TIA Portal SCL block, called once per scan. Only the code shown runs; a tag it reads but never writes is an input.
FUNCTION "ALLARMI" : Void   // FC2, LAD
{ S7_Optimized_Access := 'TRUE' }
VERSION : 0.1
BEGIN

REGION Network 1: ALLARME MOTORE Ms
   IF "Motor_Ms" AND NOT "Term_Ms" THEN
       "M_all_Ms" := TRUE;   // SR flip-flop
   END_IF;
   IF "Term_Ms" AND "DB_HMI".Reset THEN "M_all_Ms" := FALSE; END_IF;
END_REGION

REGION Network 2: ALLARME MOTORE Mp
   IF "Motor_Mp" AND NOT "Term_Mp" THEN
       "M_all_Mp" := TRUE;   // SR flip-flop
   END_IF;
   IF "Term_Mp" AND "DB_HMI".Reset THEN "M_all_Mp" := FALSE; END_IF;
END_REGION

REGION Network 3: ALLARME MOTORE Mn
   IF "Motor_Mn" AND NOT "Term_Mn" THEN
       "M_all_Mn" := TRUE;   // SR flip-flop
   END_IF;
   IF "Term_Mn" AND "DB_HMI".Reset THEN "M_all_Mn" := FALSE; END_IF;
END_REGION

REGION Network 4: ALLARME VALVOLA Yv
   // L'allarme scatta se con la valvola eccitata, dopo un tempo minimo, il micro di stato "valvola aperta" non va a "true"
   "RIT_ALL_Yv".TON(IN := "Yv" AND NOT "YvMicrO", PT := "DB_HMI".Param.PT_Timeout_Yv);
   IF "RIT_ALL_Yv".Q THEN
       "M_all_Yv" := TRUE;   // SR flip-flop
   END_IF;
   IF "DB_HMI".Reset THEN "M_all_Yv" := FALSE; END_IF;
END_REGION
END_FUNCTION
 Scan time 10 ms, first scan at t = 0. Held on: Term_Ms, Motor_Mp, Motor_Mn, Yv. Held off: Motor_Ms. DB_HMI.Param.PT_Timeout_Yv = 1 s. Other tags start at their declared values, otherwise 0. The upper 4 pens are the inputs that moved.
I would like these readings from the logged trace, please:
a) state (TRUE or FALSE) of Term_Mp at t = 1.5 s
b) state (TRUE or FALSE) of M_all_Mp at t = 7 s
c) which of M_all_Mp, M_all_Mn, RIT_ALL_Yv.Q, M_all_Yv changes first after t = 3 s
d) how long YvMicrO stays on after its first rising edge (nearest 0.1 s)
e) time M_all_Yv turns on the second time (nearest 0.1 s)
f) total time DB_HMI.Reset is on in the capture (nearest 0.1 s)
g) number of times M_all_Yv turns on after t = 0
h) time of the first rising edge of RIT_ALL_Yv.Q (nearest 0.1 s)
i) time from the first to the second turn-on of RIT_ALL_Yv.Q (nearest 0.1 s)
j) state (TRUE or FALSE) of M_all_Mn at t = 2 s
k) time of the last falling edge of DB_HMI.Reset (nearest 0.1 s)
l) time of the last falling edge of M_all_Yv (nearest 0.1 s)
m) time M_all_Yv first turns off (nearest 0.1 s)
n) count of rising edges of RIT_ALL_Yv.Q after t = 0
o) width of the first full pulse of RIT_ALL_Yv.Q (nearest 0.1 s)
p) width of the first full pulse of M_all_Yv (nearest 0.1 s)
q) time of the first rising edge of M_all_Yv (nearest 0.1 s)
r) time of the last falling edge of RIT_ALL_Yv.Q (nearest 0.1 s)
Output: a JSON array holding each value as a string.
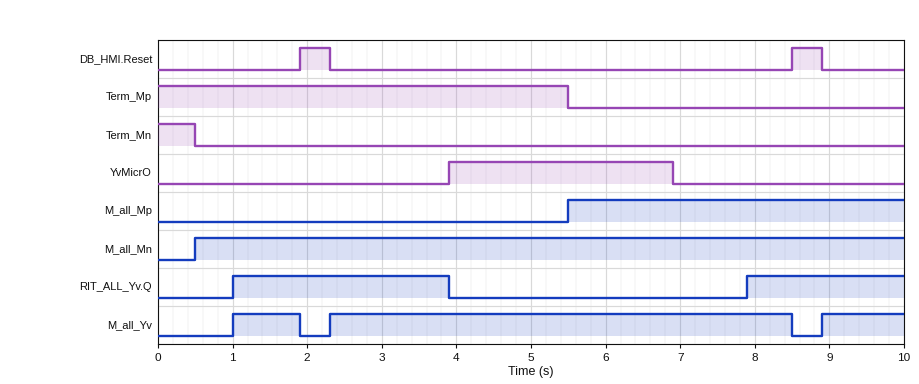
["TRUE", "TRUE", "RIT_ALL_Yv.Q", "3.0 s", "2.3 s", "0.8 s", "3", "1.0 s", "6.9 s", "TRUE", "8.9 s", "8.5 s", "1.9 s", "2", "2.9 s", "0.9 s", "1.0 s", "3.9 s"]
